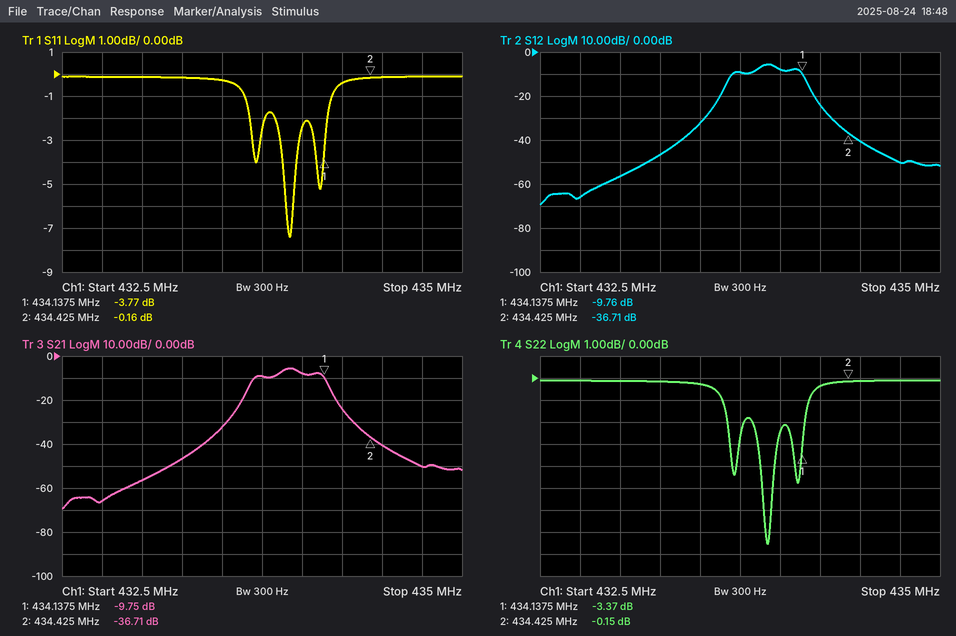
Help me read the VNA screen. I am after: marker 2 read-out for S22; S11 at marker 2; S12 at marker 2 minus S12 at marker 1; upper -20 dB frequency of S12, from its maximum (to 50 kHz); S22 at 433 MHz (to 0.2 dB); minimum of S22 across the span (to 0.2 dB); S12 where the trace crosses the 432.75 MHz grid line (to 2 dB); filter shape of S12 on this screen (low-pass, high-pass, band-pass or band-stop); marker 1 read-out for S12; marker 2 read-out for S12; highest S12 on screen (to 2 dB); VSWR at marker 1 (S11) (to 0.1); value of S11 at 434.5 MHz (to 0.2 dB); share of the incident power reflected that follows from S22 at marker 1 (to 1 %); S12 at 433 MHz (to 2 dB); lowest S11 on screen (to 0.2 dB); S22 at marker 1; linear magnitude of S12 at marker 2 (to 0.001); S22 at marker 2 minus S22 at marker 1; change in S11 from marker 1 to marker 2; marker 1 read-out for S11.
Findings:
-0.15 dB
-0.16 dB
-26.95 dB
434.25 MHz
-0.2 dB
-7.6 dB
-66 dB
band-pass
-9.76 dB
-36.71 dB
-6 dB
4.7
-0.2 dB
46 %
-56 dB
-7.4 dB
-3.37 dB
0.015
3.22 dB
3.61 dB
-3.77 dB
